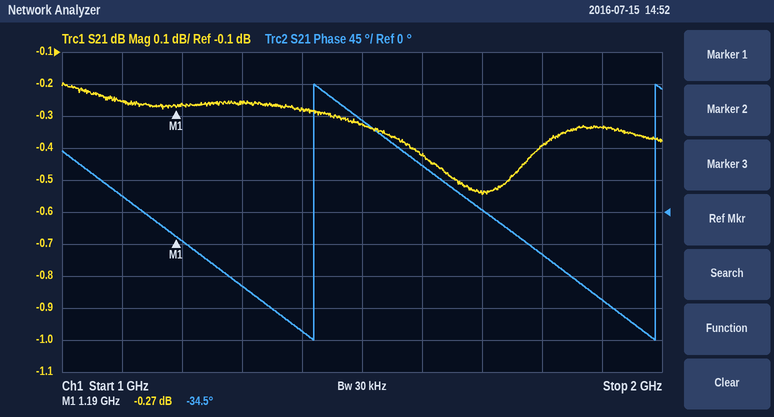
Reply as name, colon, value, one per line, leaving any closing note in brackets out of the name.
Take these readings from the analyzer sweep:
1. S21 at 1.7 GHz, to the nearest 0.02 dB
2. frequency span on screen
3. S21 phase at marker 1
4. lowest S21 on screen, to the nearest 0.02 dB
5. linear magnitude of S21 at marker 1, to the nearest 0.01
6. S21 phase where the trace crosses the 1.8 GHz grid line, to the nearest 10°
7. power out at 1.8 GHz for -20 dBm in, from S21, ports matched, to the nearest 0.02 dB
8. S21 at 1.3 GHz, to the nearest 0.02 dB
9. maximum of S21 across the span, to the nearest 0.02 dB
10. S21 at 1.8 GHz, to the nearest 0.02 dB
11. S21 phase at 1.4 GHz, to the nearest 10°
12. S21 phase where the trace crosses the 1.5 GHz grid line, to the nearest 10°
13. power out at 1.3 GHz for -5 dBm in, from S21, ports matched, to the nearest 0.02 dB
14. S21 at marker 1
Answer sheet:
S21 at 1.7 GHz, to the nearest 0.02 dB: -0.54 dB
frequency span on screen: 1 GHz
S21 phase at marker 1: -34.5°
lowest S21 on screen, to the nearest 0.02 dB: -0.54 dB
linear magnitude of S21 at marker 1, to the nearest 0.01: 0.97
S21 phase where the trace crosses the 1.8 GHz grid line, to the nearest 10°: -60°
power out at 1.8 GHz for -20 dBm in, from S21, ports matched, to the nearest 0.02 dB: -20.40 dBm
S21 at 1.3 GHz, to the nearest 0.02 dB: -0.26 dB
maximum of S21 across the span, to the nearest 0.02 dB: -0.20 dB
S21 at 1.8 GHz, to the nearest 0.02 dB: -0.40 dB
S21 phase at 1.4 GHz, to the nearest 10°: -170°
S21 phase where the trace crosses the 1.5 GHz grid line, to the nearest 10°: 130°
power out at 1.3 GHz for -5 dBm in, from S21, ports matched, to the nearest 0.02 dB: -5.26 dBm
S21 at marker 1: -0.27 dB
